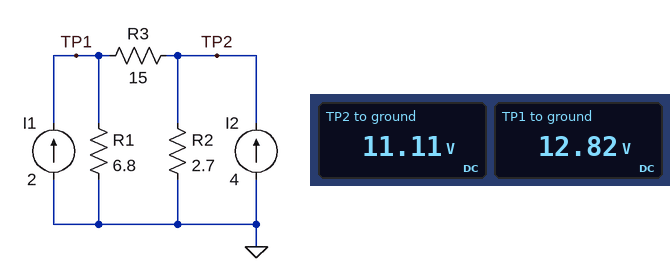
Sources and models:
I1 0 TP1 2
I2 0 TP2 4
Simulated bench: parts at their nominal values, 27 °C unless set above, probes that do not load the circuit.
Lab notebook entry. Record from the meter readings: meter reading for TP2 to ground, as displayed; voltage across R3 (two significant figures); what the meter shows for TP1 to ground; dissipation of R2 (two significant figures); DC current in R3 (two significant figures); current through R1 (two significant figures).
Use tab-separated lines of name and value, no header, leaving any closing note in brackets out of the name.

meter reading for TP2 to ground, as displayed	11.11 V
voltage across R3	1.7 V
what the meter shows for TP1 to ground	12.82 V
dissipation of R2	46 W
DC current in R3	110 mA
current through R1	1.9 A
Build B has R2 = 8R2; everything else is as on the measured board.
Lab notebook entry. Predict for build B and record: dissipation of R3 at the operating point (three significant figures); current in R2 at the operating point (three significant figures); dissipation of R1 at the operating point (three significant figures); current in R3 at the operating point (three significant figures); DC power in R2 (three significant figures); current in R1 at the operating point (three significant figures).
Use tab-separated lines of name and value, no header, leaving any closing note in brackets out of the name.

dissipation of R3 at the operating point	6.14 W
current in R2 at the operating point	3.36 A
dissipation of R1 at the operating point	47.4 W
current in R3 at the operating point	640 mA
DC power in R2	92.6 W
current in R1 at the operating point	2.64 A
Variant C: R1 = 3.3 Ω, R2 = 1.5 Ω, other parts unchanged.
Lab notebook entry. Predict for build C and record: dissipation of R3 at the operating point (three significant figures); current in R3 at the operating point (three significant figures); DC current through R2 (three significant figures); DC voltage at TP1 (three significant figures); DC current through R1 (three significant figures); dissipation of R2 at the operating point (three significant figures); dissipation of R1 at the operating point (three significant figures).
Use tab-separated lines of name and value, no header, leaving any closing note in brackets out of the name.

dissipation of R3 at the operating point	13.8 mW
current in R3 at the operating point	30.3 mA
DC current through R2	4.03 A
DC voltage at TP1	6.50 V
DC current through R1	1.97 A
dissipation of R2 at the operating point	24.4 W
dissipation of R1 at the operating point	12.8 W
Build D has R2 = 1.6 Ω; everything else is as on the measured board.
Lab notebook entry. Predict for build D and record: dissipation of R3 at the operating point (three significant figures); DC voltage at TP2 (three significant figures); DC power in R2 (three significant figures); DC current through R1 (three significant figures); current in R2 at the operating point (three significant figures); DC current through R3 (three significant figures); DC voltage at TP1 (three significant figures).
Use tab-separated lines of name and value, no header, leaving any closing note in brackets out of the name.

dissipation of R3 at the operating point	1.42 W
DC voltage at TP2	6.89 V
DC power in R2	29.7 W
DC current through R1	1.69 A
current in R2 at the operating point	4.31 A
DC current through R3	308 mA
DC voltage at TP1	11.5 V
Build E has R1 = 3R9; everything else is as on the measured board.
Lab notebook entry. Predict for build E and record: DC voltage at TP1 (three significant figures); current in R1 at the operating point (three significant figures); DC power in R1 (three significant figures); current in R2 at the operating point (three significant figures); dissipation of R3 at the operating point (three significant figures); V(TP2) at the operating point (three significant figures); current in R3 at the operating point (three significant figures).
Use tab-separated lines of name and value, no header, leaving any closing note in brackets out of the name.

DC voltage at TP1	8.34 V
current in R1 at the operating point	2.14 A
DC power in R1	17.8 W
current in R2 at the operating point	3.86 A
dissipation of R3 at the operating point	289 mW
V(TP2) at the operating point	10.4 V
current in R3 at the operating point	139 mA
